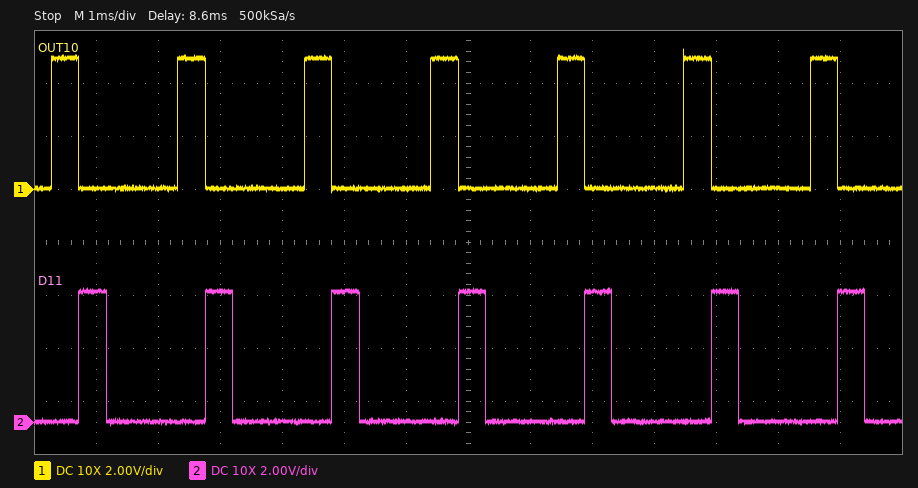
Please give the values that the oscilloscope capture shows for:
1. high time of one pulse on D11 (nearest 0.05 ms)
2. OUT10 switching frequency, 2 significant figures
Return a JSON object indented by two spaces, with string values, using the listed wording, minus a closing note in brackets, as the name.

{
  "high time of one pulse on D11": "0.45 ms",
  "OUT10 switching frequency, 2 significant figures": "490 Hz"
}
